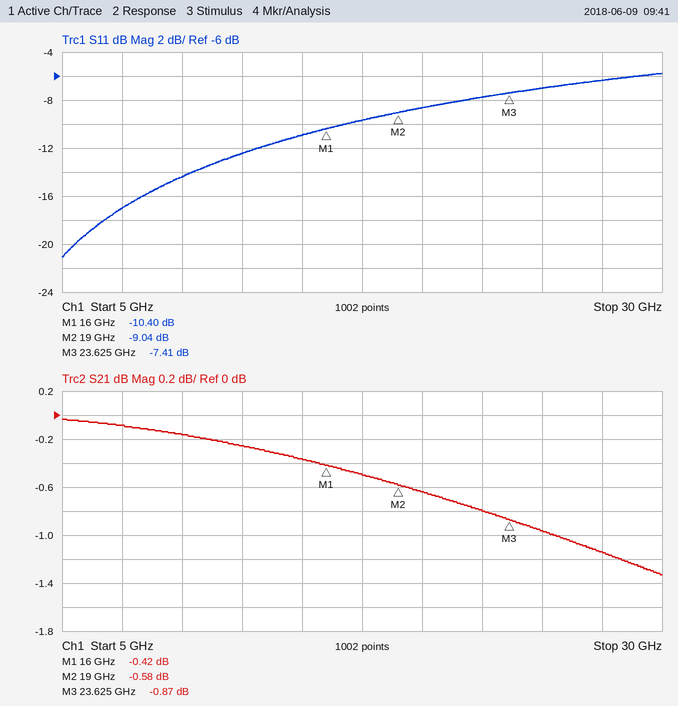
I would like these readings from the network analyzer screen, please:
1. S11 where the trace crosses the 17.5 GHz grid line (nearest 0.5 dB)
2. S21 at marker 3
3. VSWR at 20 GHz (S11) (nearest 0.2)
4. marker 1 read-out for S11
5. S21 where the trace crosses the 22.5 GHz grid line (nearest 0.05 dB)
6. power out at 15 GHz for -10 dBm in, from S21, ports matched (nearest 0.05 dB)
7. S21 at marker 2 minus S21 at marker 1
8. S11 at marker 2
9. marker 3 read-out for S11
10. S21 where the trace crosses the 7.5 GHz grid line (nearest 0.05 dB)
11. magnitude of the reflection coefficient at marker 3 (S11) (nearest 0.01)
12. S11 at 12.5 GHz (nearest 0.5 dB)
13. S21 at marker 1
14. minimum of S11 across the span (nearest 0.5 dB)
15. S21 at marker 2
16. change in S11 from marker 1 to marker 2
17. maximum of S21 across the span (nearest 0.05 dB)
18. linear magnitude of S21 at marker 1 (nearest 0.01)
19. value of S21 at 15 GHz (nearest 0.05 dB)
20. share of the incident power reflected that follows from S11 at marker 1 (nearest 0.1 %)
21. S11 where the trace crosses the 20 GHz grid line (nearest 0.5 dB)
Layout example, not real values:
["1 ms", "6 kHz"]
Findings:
["-9.5 dB", "-0.87 dB", "2.2", "-10.40 dB", "-0.80 dB", "-10.35 dBm", "-0.16 dB", "-9.04 dB", "-7.41 dB", "-0.10 dB", "0.43", "-12.5 dB", "-0.42 dB", "-21.0 dB", "-0.58 dB", "1.36 dB", "-0.05 dB", "0.95", "-0.35 dB", "9.1 %", "-8.5 dB"]
